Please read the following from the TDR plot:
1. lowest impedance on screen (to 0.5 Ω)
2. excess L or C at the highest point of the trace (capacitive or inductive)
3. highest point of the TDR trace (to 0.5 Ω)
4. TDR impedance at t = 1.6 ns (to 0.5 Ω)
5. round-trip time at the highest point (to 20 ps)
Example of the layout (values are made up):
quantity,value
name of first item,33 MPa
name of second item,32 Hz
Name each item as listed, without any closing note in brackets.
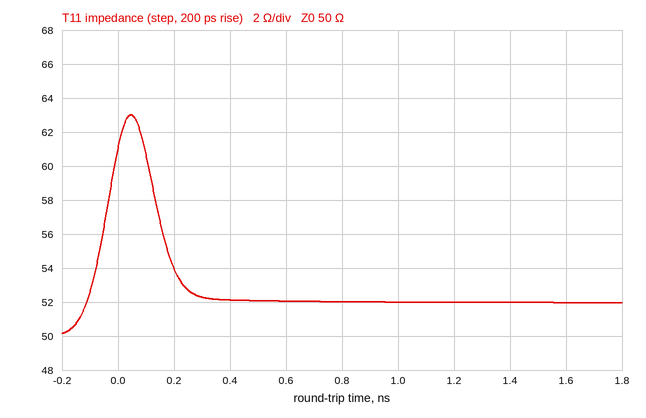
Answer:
quantity,value
lowest impedance on screen,50.0 Ω
excess L or C at the highest point of the trace,inductive
highest point of the TDR trace,63.0 Ω
TDR impedance at t = 1.6 ns,52.0 Ω
round-trip time at the highest point,40 ps
